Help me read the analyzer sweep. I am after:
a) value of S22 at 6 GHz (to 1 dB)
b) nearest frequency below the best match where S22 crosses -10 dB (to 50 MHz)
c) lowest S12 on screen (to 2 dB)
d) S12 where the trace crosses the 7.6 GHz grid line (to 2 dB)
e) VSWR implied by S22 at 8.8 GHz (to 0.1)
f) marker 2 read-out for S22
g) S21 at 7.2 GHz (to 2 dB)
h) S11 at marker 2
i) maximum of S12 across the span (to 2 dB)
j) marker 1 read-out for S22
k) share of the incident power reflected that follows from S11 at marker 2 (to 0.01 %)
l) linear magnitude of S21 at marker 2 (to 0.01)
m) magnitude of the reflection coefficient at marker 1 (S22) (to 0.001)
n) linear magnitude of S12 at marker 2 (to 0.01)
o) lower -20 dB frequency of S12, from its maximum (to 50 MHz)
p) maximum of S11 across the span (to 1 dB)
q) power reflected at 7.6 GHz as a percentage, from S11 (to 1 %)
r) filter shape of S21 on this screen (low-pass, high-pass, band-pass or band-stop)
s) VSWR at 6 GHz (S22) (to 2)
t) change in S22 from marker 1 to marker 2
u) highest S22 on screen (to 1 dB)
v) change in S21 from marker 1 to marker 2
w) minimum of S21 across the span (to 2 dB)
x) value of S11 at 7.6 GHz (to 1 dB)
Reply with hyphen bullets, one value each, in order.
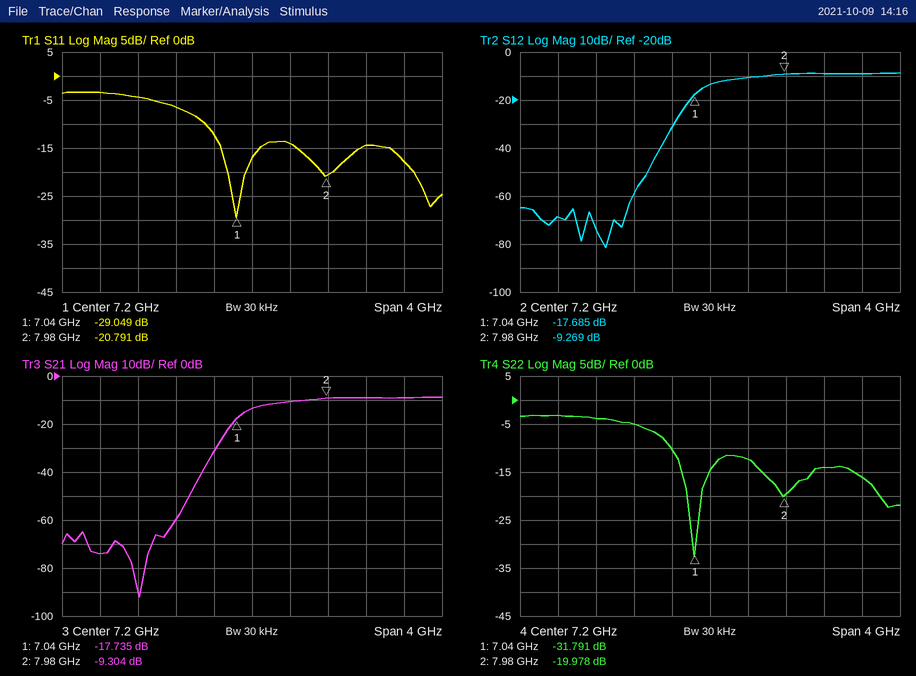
- -4 dB
- 6.80 GHz
- -82 dB
- -10 dB
- 1.4
- -19.978 dB
- -14 dB
- -20.791 dB
- -8 dB
- -31.791 dB
- 0.83 %
- 0.34
- 0.026
- 0.34
- 6.85 GHz
- -3 dB
- 4 %
- high-pass
- 4
- 11.813 dB
- -3 dB
- 8.431 dB
- -92 dB
- -14 dB
